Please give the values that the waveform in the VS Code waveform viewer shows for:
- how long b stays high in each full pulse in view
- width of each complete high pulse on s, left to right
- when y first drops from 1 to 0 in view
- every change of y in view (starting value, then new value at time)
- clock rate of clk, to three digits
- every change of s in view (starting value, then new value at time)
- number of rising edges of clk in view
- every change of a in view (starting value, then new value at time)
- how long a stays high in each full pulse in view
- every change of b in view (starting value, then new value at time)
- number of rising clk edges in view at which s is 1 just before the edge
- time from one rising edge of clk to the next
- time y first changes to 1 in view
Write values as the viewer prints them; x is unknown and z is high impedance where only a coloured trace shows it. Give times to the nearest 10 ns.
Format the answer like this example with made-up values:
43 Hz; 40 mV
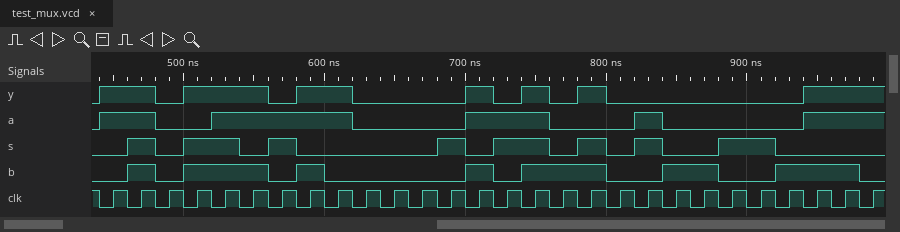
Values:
20 ns, 60 ns, 20 ns, 20 ns, 60 ns, 40 ns, 60 ns; 20 ns, 40 ns, 20 ns, 20 ns, 40 ns, 20 ns, 20 ns, 40 ns; 480 ns; 0, 1 at 440 ns, 0 at 480 ns, 1 at 500 ns, 0 at 560 ns, 1 at 580 ns, 0 at 620 ns, 1 at 700 ns, 0 at 720 ns, 1 at 740 ns, 0 at 760 ns, 1 at 780 ns, 0 at 800 ns, 1 at 940 ns; 50.0 MHz; 0, 1 at 460 ns, 0 at 480 ns, 1 at 500 ns, 0 at 540 ns, 1 at 560 ns, 0 at 580 ns, 1 at 680 ns, 0 at 700 ns, 1 at 720 ns, 0 at 760 ns, 1 at 780 ns, 0 at 800 ns, 1 at 820 ns, 0 at 840 ns, 1 at 880 ns, 0 at 920 ns; 28; 0, 1 at 440 ns, 0 at 480 ns, 1 at 520 ns, 0 at 620 ns, 1 at 700 ns, 0 at 760 ns, 1 at 820 ns, 0 at 840 ns, 1 at 940 ns; 40 ns, 100 ns, 60 ns, 20 ns; 0, 1 at 460 ns, 0 at 480 ns, 1 at 500 ns, 0 at 560 ns, 1 at 580 ns, 0 at 600 ns, 1 at 700 ns, 0 at 720 ns, 1 at 740 ns, 0 at 800 ns, 1 at 840 ns, 0 at 880 ns, 1 at 920 ns, 0 at 980 ns; 11; 20 ns; 440 ns
